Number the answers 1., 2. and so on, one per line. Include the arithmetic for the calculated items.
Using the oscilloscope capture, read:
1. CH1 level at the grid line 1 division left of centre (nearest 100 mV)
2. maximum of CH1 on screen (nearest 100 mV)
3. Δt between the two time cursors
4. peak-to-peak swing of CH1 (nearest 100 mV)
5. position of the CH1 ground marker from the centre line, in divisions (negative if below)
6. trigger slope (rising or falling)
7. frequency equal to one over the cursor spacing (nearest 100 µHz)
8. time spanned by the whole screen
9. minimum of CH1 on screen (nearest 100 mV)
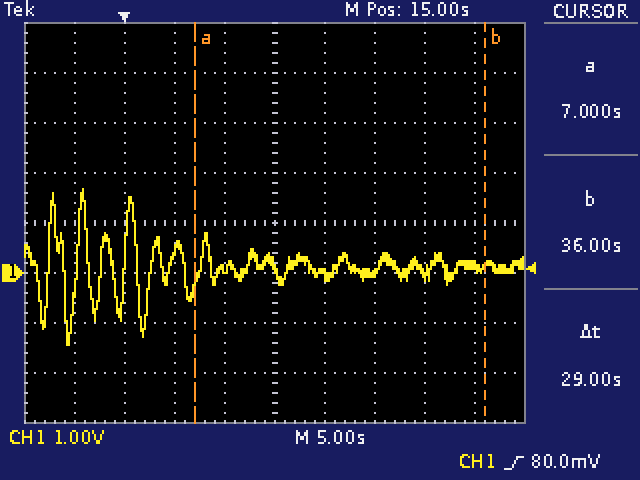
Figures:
1. 100 mV
2. 1.7 V
3. 29 s
4. 1.7 V − (-1.4 V) = 3.1 V
5. -1.0 div
6. rising
7. 1 / 29 s ≈ 34.5 mHz
8. 50 s
9. -1.4 V
